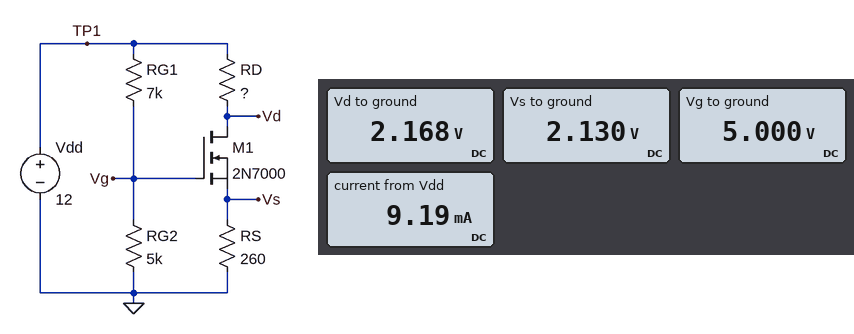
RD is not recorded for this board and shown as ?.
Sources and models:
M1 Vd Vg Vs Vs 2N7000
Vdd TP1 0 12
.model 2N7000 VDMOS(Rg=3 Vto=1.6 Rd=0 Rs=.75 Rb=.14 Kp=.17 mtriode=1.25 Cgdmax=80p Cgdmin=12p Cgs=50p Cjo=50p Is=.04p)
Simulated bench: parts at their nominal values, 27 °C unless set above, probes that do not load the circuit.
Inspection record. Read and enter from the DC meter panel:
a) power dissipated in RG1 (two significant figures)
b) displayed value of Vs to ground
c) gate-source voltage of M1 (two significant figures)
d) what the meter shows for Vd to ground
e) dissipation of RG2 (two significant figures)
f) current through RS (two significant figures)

7.0 mW
2.130 V
2.9 V
2.168 V
5.0 mW
8.2 mA
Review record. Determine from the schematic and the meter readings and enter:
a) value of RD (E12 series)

1.2 kΩ
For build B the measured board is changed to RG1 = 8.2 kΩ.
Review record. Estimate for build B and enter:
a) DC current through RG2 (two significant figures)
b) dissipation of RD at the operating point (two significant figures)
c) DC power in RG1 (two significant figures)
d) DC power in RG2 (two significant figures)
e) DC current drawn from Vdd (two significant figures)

910 µA
80 mW
6.8 mW
4.1 mW
9.1 mA
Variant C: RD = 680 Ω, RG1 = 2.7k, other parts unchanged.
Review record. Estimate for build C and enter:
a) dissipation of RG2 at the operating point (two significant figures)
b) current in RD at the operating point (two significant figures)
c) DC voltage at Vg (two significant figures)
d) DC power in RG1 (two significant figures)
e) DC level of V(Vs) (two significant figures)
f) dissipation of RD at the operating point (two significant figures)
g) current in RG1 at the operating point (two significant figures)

12 mW
13 mA
7.8 V
6.6 mW
3.3 V
110 mW
1.6 mA
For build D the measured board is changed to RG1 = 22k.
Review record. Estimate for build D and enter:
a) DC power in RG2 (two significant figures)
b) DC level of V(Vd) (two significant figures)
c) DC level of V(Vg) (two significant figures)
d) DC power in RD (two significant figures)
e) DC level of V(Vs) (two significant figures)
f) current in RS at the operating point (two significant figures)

990 µW
9.7 V
2.2 V
4.4 mW
500 mV
1.9 mA
